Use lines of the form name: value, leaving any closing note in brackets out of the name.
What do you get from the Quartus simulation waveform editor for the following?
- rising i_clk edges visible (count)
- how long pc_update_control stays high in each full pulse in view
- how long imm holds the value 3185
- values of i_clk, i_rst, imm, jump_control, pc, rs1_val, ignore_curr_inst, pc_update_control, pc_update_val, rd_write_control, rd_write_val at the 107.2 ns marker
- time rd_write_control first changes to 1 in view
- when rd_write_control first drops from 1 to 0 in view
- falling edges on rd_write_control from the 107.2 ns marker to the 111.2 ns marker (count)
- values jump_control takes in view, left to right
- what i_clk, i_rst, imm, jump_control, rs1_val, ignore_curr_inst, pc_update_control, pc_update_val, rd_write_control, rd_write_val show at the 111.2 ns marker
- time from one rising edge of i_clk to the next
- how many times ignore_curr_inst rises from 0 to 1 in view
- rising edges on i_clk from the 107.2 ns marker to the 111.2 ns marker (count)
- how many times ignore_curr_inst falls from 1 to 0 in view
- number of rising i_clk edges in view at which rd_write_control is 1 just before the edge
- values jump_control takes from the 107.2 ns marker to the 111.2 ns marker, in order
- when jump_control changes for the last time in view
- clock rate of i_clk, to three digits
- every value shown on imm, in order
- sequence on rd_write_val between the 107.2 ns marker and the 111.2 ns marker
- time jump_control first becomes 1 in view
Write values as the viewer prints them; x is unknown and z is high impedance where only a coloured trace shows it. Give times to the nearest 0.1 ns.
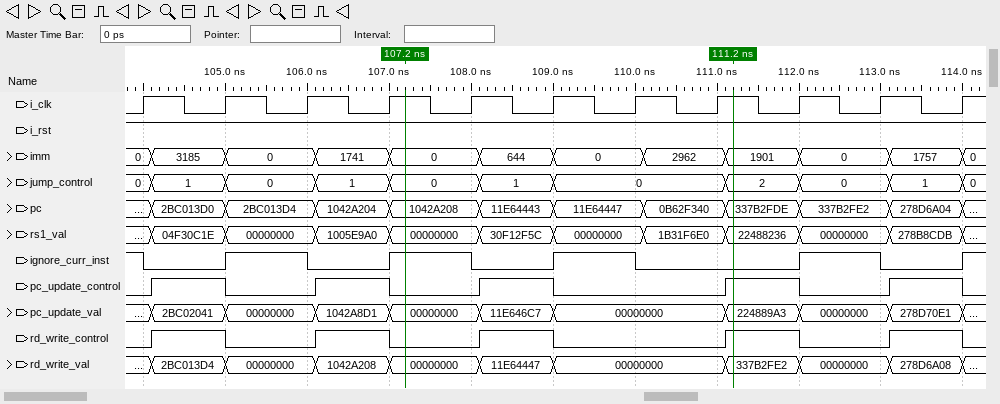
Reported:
rising i_clk edges visible: 11
how long pc_update_control stays high in each full pulse in view: 0.9 ns, 0.9 ns, 0.9 ns, 0.9 ns, 0.9 ns
how long imm holds the value 3185: 0.9 ns
values of i_clk, i_rst, imm, jump_control, pc, rs1_val, ignore_curr_inst, pc_update_control, pc_update_val, rd_write_control, rd_write_val at the 107.2 ns marker: i_clk=1, i_rst=1, imm=0, jump_control=0, pc=1042A208, rs1_val=00000000, ignore_curr_inst=1, pc_update_control=0, pc_update_val=00000000, rd_write_control=0, rd_write_val=00000000
time rd_write_control first changes to 1 in view: 104.1 ns
when rd_write_control first drops from 1 to 0 in view: 105 ns
falling edges on rd_write_control from the 107.2 ns marker to the 111.2 ns marker: 1
values jump_control takes in view, left to right: 0, 1, 0, 1, 0, 1, 0, 2, 0, 1, 0
what i_clk, i_rst, imm, jump_control, rs1_val, ignore_curr_inst, pc_update_control, pc_update_val, rd_write_control, rd_write_val show at the 111.2 ns marker: i_clk=1, i_rst=1, imm=1901, jump_control=2, rs1_val=22488236, ignore_curr_inst=0, pc_update_control=1, pc_update_val=224889A3, rd_write_control=1, rd_write_val=337B2FE2
time from one rising edge of i_clk to the next: 1 ns
how many times ignore_curr_inst rises from 0 to 1 in view: 5
rising edges on i_clk from the 107.2 ns marker to the 111.2 ns marker: 4
how many times ignore_curr_inst falls from 1 to 0 in view: 5
number of rising i_clk edges in view at which rd_write_control is 1 just before the edge: 5
values jump_control takes from the 107.2 ns marker to the 111.2 ns marker, in order: 0, 1, 0, 2
when jump_control changes for the last time in view: 114 ns
clock rate of i_clk, to three digits: 1.00 GHz
every value shown on imm, in order: 0, 3185, 0, 1741, 0, 644, 0, 2962, 1901, 0, 1757, 0
sequence on rd_write_val between the 107.2 ns marker and the 111.2 ns marker: 00000000, 11E64447, 00000000, 337B2FE2
time jump_control first becomes 1 in view: 104.1 ns
